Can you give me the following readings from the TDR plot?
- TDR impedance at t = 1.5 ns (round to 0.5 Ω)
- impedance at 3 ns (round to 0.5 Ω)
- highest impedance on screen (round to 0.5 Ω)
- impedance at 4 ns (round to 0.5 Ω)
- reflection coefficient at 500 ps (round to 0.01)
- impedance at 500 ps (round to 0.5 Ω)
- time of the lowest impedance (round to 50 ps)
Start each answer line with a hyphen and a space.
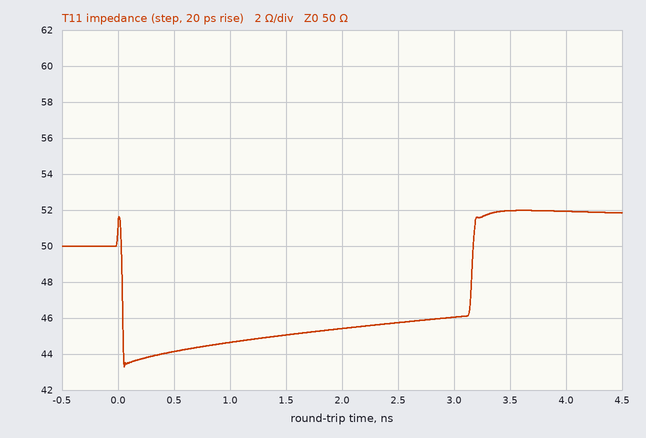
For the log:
- 45.0 Ω
- 46.0 Ω
- 52.0 Ω
- 52.0 Ω
- -0.06
- 44.0 Ω
- 50 ps
